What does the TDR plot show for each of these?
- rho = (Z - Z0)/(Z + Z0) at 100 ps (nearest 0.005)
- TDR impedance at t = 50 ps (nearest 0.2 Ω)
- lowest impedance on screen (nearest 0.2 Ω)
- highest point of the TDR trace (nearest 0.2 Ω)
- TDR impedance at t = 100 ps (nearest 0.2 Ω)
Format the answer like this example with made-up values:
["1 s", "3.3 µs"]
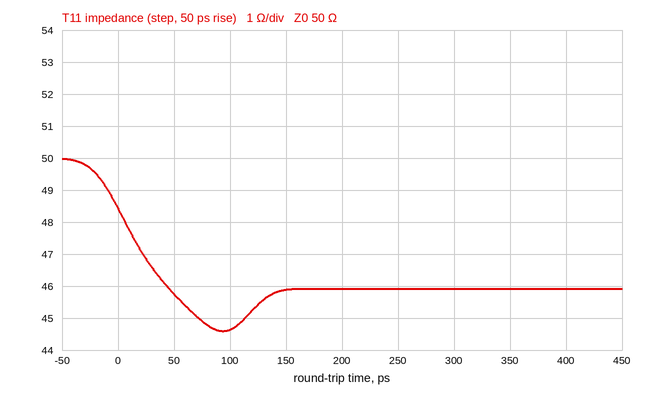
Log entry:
["-0.055", "45.8 Ω", "44.6 Ω", "50.0 Ω", "44.6 Ω"]
